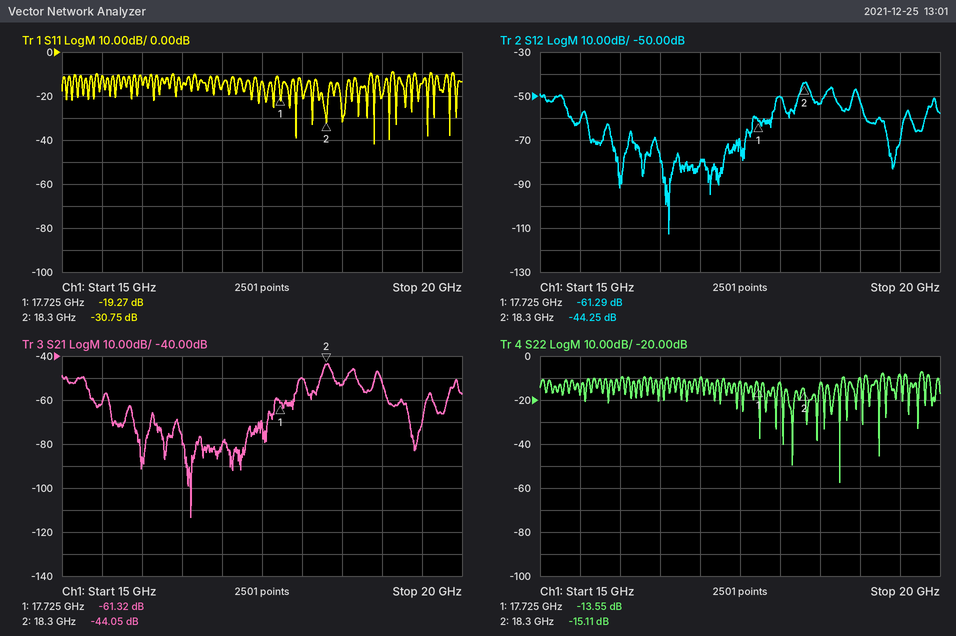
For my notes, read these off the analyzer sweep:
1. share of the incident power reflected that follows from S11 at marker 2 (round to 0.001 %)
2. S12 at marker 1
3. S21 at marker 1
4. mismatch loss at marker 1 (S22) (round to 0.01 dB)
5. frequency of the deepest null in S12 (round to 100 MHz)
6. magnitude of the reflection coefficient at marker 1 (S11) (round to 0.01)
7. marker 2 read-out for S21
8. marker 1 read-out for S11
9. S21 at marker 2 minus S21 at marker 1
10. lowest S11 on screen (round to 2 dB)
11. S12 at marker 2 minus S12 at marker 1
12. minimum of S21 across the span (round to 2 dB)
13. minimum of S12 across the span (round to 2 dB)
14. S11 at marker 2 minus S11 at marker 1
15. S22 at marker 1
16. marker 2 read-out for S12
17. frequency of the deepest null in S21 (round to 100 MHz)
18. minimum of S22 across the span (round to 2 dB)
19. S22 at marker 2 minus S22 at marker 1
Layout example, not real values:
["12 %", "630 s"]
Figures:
["0.084 %", "-61.29 dB", "-61.32 dB", "0.20 dB", "16.6 GHz", "0.11", "-44.05 dB", "-19.27 dB", "17.27 dB", "-42 dB", "17.04 dB", "-114 dB", "-112 dB", "-11.48 dB", "-13.55 dB", "-44.25 dB", "16.6 GHz", "-58 dB", "-1.56 dB"]
